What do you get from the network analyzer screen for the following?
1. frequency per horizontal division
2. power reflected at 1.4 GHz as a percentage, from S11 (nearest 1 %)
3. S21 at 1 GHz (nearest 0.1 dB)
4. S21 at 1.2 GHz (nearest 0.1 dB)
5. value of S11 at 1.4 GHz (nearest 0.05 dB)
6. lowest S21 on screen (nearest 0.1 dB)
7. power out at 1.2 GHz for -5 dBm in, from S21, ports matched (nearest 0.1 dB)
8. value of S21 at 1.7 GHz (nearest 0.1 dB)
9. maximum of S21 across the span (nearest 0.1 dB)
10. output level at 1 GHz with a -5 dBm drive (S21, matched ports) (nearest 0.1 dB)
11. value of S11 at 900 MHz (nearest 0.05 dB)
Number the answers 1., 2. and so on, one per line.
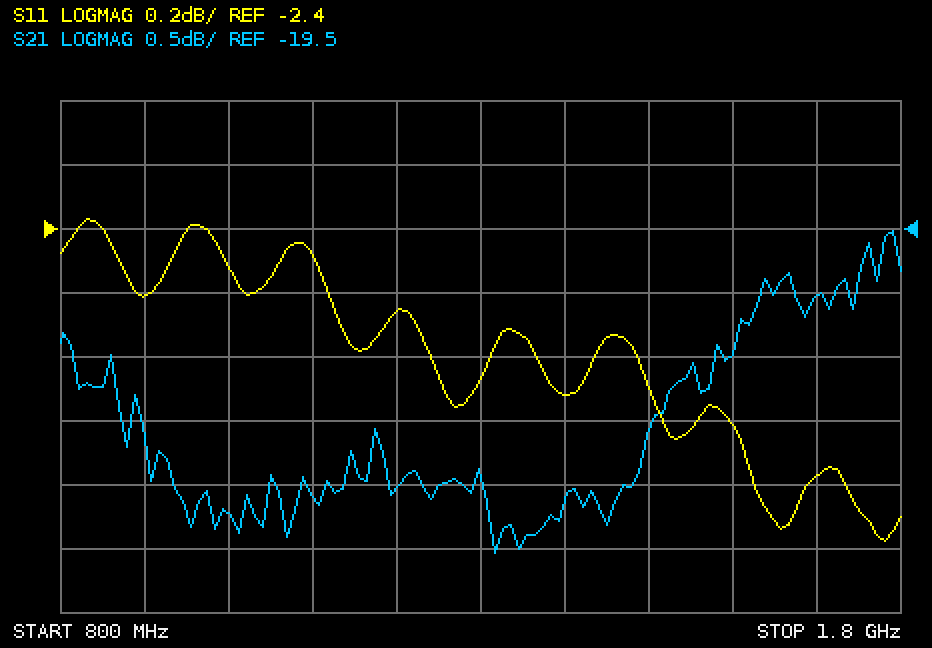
1. 100 MHz
2. 51 %
3. -21.7 dB
4. -21.5 dB
5. -2.90 dB
6. -22.0 dB
7. -26.5 dBm
8. -20.0 dB
9. -19.5 dB
10. -26.7 dBm
11. -2.60 dB
